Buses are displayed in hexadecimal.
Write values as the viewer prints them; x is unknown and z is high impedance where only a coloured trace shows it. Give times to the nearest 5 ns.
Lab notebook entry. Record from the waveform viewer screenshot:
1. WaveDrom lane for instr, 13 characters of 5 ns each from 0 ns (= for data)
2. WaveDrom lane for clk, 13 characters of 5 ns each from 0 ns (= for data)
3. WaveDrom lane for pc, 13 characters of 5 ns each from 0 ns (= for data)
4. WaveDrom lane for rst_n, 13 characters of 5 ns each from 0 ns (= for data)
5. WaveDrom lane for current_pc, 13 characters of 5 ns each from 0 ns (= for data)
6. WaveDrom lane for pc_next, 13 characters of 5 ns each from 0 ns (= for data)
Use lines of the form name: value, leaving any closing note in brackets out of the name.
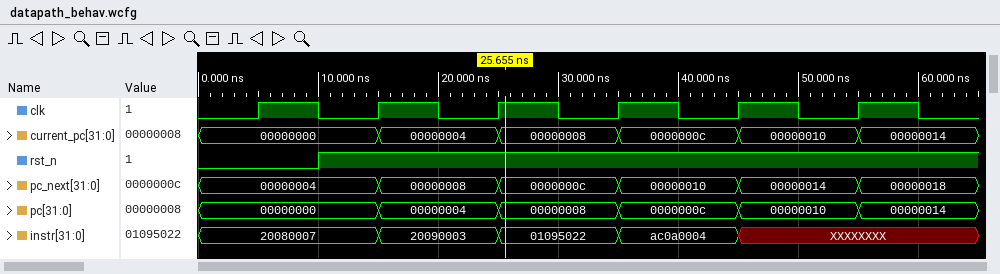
WaveDrom lane for instr, 13 characters of 5 ns each from 0 ns: {name: 'instr', wave: '=..=.=.=.x...', data: '20080007 20090003 01095022 ac0a0004'}
WaveDrom lane for clk, 13 characters of 5 ns each from 0 ns: {name: 'clk', wave: '0101010101010'}
WaveDrom lane for pc, 13 characters of 5 ns each from 0 ns: {name: 'pc', wave: '=..=.=.=.=.=.', data: '00000000 00000004 00000008 0000000c 00000010 00000014'}
WaveDrom lane for rst_n, 13 characters of 5 ns each from 0 ns: {name: 'rst_n', wave: '0.1..........'}
WaveDrom lane for current_pc, 13 characters of 5 ns each from 0 ns: {name: 'current_pc', wave: '=..=.=.=.=.=.', data: '00000000 00000004 00000008 0000000c 00000010 00000014'}
WaveDrom lane for pc_next, 13 characters of 5 ns each from 0 ns: {name: 'pc_next', wave: '=..=.=.=.=.=.', data: '00000004 00000008 0000000c 00000010 00000014 00000018'}
